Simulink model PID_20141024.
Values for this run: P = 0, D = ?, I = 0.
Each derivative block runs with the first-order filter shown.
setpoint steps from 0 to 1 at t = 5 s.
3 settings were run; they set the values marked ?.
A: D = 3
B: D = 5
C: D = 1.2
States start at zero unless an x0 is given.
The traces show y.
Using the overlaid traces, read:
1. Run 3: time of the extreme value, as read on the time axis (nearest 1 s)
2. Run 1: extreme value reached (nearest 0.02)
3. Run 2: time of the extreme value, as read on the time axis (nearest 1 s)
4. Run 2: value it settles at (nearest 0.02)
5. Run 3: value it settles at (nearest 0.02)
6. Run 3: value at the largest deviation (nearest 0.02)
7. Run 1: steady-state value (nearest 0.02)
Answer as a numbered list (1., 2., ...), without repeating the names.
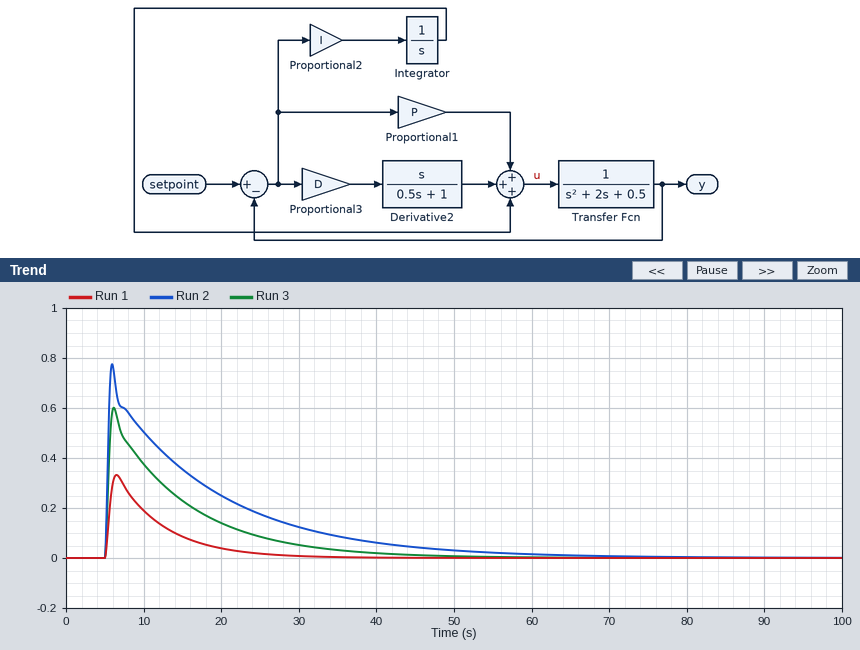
1. 6 s
2. 0.34
3. 6 s
4. 0.00
5. 0.00
6. 0.60
7. 0.00
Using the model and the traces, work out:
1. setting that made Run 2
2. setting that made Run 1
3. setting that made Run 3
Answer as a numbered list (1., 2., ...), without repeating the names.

1. B
2. C
3. A
